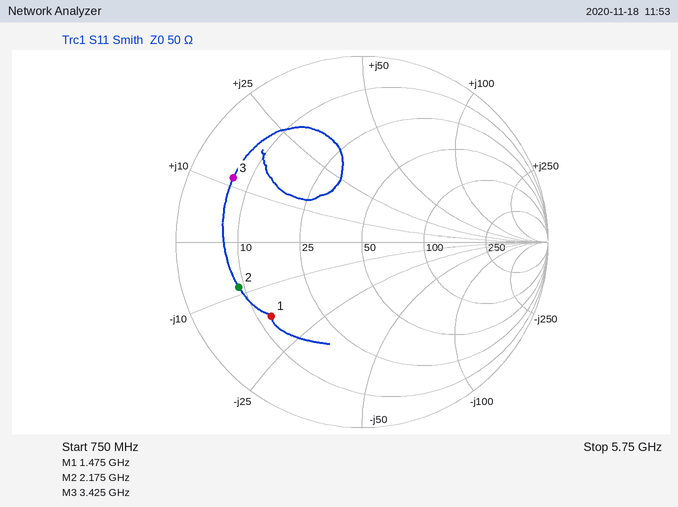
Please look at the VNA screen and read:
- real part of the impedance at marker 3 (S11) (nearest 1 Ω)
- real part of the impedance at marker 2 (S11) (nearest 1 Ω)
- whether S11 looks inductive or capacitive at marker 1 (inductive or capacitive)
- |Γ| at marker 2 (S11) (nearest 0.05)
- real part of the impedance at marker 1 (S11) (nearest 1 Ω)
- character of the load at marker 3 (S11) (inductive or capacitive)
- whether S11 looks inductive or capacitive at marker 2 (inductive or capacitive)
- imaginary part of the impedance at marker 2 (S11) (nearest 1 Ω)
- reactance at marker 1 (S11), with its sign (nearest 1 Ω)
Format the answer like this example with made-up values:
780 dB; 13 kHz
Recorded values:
7 Ω; 9 Ω; capacitive; 0.70; 13 Ω; inductive; capacitive; -9 Ω; -17 Ω
